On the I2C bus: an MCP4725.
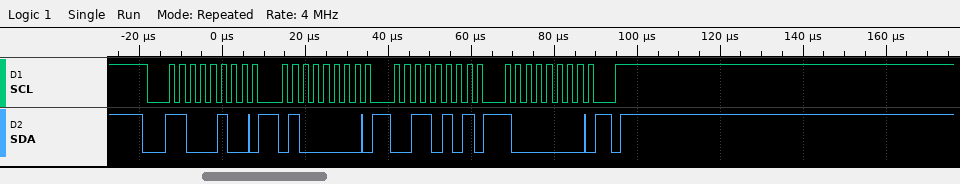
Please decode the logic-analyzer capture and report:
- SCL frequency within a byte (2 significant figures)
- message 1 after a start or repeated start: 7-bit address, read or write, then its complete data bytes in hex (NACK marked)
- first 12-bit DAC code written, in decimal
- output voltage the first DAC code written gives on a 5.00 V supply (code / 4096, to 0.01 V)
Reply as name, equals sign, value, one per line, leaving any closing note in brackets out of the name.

SCL frequency within a byte = 400 kHz
message 1 after a start or repeated start: 7-bit address, read or write, then its complete data bytes in hex = 0x62 write: 40 35 80
first 12-bit DAC code written, in decimal = 856
output voltage the first DAC code written gives on a 5.00 V supply = 1.04 V
